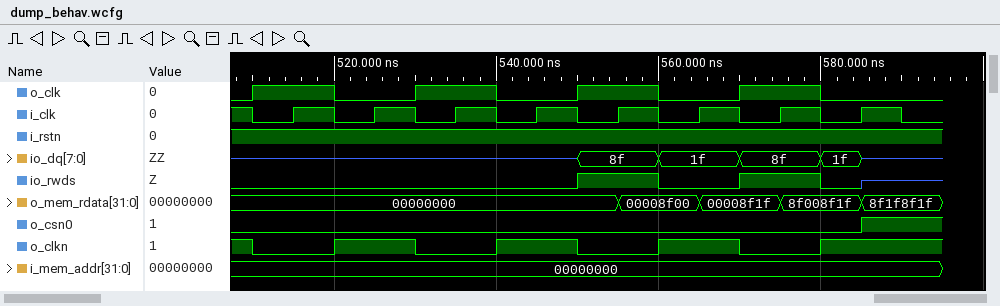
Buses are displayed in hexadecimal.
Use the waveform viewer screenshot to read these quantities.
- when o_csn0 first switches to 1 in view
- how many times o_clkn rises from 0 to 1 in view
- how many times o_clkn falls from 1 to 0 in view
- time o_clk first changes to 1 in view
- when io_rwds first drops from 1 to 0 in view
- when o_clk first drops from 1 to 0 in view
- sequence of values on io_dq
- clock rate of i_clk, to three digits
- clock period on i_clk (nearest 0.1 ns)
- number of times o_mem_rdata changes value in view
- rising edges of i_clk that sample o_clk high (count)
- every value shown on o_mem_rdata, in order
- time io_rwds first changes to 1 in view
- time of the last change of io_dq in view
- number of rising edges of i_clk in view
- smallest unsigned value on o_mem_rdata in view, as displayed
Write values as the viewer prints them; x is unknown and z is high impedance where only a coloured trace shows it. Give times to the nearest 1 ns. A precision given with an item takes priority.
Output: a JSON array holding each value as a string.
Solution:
["585 ns", "4", "4", "510 ns", "560 ns", "520 ns", "z, 8f, 1f, 8f, 1f, z", "100 MHz", "10 ns", "4", "4", "00000000, 00008f00, 00008f1f, 8f008f1f, 8f1f8f1f", "550 ns", "585 ns", "8", "00000000"]
